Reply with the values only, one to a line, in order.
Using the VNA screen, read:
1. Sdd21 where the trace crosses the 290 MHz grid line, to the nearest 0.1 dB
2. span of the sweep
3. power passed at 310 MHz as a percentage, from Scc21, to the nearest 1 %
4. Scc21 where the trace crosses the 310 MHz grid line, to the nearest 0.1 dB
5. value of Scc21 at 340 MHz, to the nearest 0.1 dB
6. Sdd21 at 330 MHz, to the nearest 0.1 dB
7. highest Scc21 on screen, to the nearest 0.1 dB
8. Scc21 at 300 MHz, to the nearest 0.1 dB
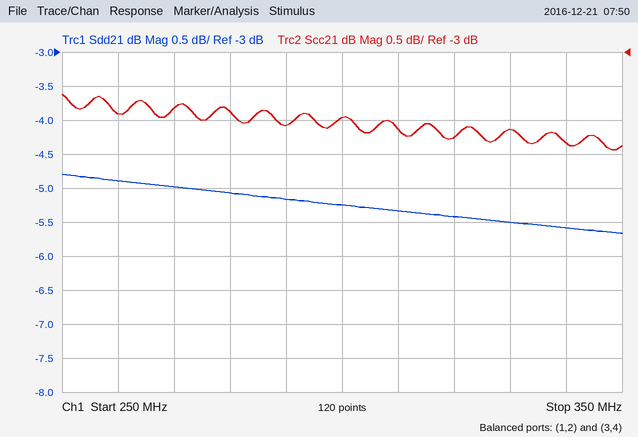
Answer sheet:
-5.2 dB
100 MHz
39 %
-4.1 dB
-4.3 dB
-5.5 dB
-3.6 dB
-4.0 dB
